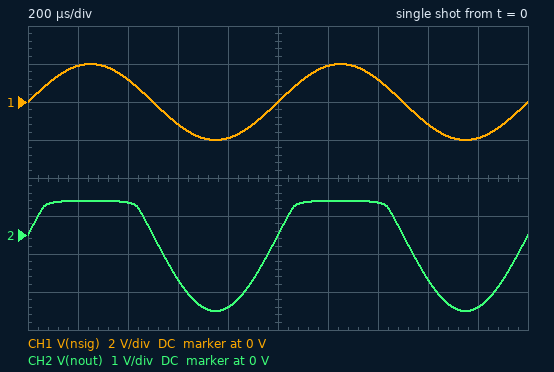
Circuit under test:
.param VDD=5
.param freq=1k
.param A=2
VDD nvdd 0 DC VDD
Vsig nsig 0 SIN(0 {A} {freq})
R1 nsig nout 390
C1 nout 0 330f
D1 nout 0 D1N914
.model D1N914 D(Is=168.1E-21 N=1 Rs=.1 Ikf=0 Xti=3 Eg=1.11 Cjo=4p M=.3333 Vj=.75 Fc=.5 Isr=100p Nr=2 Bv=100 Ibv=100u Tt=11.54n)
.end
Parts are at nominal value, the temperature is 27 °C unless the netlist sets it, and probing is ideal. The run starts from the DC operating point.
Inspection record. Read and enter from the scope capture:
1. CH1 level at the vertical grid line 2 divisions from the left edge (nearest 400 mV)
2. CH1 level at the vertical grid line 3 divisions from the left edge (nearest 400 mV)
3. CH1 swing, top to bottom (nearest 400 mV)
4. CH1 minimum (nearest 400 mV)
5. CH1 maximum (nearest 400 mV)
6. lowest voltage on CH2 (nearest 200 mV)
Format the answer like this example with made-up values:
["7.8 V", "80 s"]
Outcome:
["1.2 V", "-1.2 V", "4.0 V", "-2.0 V", "2.0 V", "-2.0 V"]
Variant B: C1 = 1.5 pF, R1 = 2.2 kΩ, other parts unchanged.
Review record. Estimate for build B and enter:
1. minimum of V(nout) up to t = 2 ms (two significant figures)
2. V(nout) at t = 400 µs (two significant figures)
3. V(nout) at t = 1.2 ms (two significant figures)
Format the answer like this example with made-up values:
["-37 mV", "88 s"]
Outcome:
["-2.0 V", "790 mV", "830 mV"]
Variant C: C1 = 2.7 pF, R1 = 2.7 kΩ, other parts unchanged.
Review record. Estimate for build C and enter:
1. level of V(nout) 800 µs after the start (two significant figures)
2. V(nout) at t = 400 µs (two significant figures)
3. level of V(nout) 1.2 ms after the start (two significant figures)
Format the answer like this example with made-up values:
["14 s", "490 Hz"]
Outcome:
["-1.9 V", "780 mV", "820 mV"]
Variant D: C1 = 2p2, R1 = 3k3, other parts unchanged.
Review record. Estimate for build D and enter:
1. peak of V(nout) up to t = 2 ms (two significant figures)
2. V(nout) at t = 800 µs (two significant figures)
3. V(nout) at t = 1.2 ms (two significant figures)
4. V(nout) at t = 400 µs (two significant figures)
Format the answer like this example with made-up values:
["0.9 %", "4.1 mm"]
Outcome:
["820 mV", "-1.9 V", "810 mV", "770 mV"]
